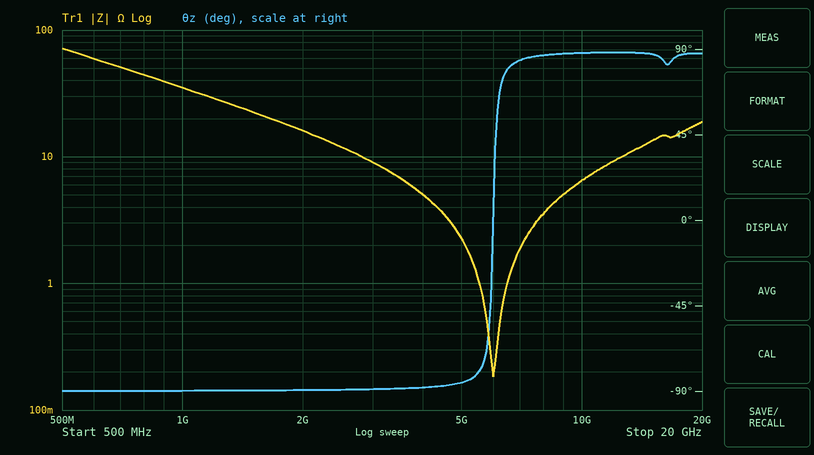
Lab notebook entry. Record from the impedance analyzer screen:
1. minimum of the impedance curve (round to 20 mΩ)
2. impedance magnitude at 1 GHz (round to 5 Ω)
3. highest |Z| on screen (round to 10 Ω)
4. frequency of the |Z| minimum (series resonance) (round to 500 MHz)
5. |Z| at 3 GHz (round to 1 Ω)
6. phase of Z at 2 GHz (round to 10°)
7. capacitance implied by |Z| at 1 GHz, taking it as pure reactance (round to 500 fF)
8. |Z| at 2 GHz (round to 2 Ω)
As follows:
180 mΩ
35 Ω
70 Ω
6.0 GHz
9 Ω
-90°
4.5 pF
16 Ω
